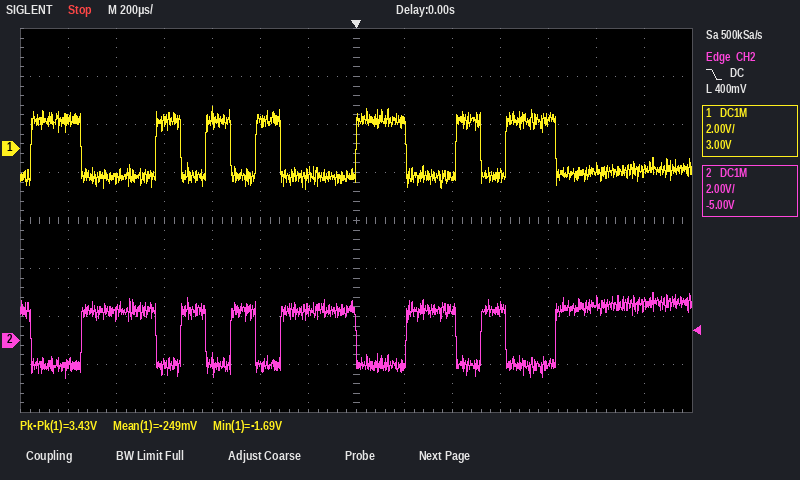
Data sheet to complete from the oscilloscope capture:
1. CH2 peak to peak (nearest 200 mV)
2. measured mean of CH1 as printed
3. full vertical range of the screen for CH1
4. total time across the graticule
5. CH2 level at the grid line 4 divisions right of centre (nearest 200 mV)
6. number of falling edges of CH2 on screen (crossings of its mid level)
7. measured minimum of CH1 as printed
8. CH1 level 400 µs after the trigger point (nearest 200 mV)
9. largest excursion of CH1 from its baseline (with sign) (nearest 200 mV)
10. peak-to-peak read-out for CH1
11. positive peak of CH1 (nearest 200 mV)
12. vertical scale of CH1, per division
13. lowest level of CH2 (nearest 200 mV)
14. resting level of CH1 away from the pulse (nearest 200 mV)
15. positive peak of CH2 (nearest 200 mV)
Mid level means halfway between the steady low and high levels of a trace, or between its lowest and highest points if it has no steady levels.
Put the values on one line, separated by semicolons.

3.6 V; -249 mV; 16 V; 2.8 ms; -1.0 V; 7; -1.69 V; -1.2 V; +2.8 V; 3.43 V; 1.8 V; 2 V; -1.6 V; -1.0 V; 2.0 V
